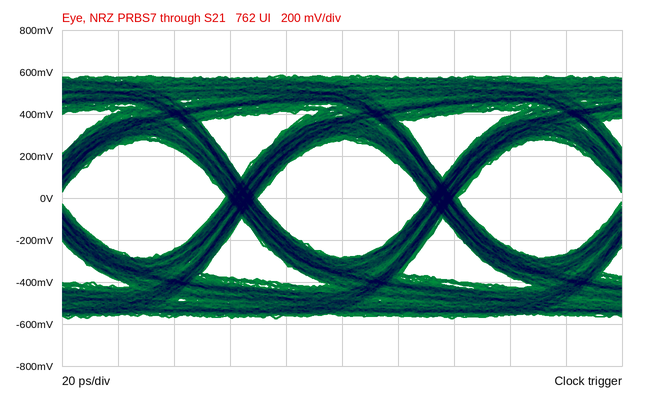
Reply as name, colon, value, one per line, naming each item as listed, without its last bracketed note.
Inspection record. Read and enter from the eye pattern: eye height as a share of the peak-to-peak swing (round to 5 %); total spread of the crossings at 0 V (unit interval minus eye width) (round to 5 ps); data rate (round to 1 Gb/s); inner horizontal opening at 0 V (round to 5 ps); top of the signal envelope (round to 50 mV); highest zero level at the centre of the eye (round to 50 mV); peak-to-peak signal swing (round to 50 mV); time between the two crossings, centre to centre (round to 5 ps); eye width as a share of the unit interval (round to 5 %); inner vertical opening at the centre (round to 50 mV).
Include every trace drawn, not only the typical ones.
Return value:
eye height as a share of the peak-to-peak swing: 50 %
total spread of the crossings at 0 V (unit interval minus eye width): 10 ps
data rate: 14 Gb/s
inner horizontal opening at 0 V: 60 ps
top of the signal envelope: 600 mV
highest zero level at the centre of the eye: -300 mV
peak-to-peak signal swing: 1.15 V
time between the two crossings, centre to centre: 70 ps
eye width as a share of the unit interval: 85 %
inner vertical opening at the centre: 550 mV
